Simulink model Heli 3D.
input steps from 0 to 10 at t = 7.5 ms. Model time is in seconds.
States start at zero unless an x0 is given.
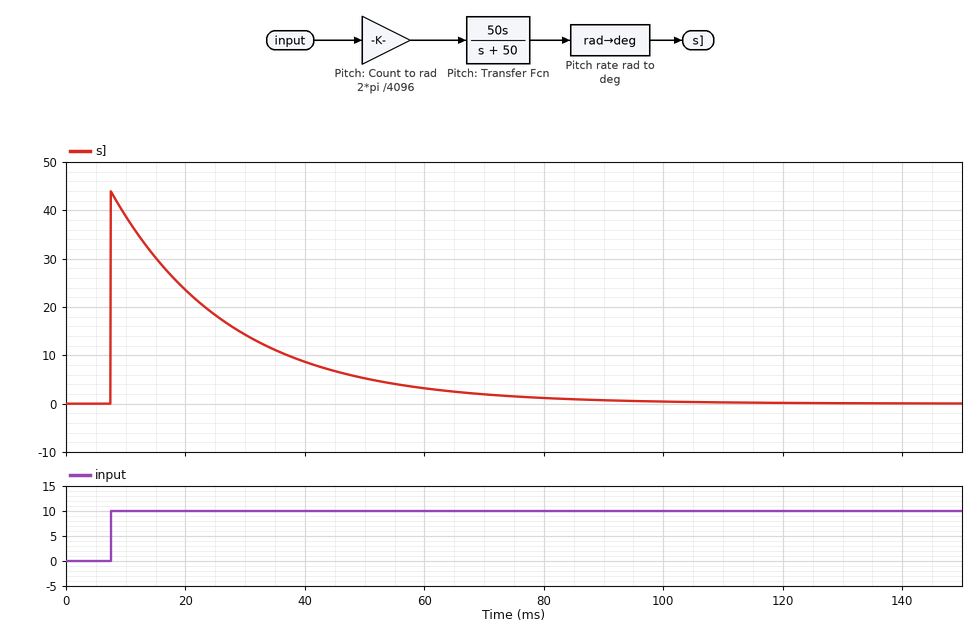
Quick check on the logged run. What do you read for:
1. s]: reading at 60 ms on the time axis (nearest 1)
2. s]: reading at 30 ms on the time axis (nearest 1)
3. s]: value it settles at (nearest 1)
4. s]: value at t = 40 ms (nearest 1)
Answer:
3
14
0
9
